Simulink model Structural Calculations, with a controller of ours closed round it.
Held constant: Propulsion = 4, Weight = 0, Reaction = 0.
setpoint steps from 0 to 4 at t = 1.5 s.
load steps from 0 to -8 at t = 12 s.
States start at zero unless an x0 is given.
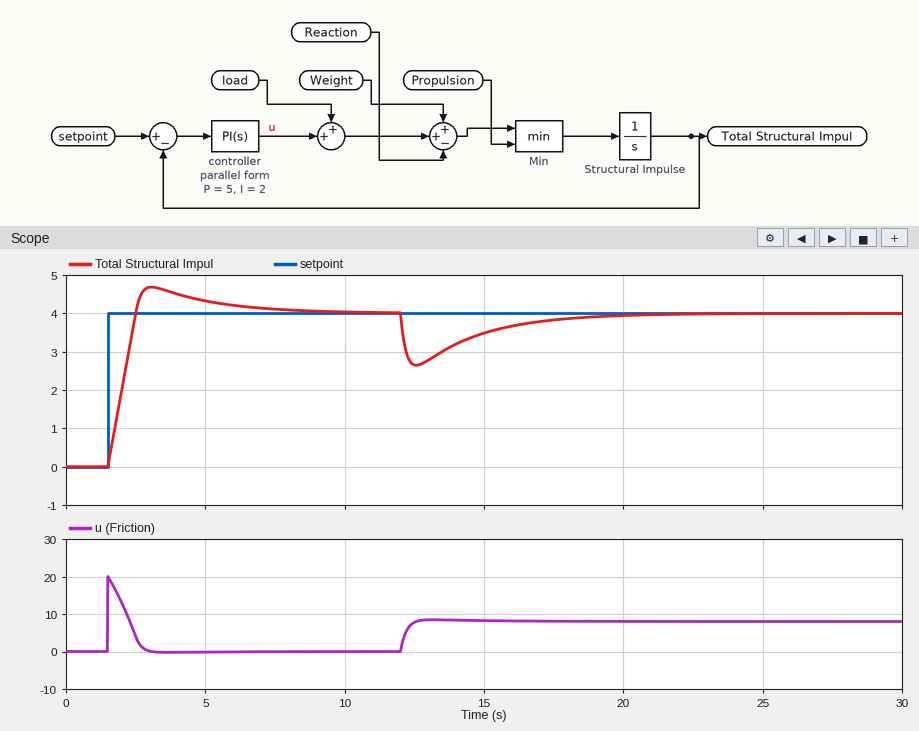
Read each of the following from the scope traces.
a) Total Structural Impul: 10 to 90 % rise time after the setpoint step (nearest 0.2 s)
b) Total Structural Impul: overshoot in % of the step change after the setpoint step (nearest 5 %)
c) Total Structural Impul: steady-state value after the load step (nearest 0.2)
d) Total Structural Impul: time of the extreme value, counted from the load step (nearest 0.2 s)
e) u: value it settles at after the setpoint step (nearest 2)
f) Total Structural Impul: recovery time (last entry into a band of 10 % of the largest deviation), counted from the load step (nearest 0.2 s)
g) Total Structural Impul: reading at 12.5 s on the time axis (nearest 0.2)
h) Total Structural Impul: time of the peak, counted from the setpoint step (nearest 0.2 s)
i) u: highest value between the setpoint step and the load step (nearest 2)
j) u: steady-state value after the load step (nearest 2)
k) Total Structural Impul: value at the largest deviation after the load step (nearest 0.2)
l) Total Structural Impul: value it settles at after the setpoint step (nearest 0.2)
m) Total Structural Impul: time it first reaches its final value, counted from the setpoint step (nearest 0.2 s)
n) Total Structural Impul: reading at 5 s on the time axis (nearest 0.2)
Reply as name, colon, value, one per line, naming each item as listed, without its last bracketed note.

Total Structural Impul: 10 to 90 % rise time after the setpoint step: 0.8 s
Total Structural Impul: overshoot in % of the step change after the setpoint step: 15 %
Total Structural Impul: steady-state value after the load step: 4.0
Total Structural Impul: time of the extreme value, counted from the load step: 0.6 s
u: value it settles at after the setpoint step: 0
Total Structural Impul: recovery time (last entry into a band of 10 % of the largest deviation), counted from the load step: 6.0 s
Total Structural Impul: reading at 12.5 s on the time axis: 2.6
Total Structural Impul: time of the peak, counted from the setpoint step: 1.6 s
u: highest value between the setpoint step and the load step: 20
u: steady-state value after the load step: 8
Total Structural Impul: value at the largest deviation after the load step: 2.6
Total Structural Impul: value it settles at after the setpoint step: 4.0
Total Structural Impul: time it first reaches its final value, counted from the setpoint step: 1.0 s
Total Structural Impul: reading at 5 s on the time axis: 4.4
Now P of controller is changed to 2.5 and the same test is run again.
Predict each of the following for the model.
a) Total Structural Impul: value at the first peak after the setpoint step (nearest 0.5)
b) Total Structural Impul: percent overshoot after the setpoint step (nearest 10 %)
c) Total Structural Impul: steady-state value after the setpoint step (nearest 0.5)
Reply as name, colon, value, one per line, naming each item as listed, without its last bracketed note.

Total Structural Impul: value at the first peak after the setpoint step: 5.0
Total Structural Impul: percent overshoot after the setpoint step: 30 %
Total Structural Impul: steady-state value after the setpoint step: 4.0
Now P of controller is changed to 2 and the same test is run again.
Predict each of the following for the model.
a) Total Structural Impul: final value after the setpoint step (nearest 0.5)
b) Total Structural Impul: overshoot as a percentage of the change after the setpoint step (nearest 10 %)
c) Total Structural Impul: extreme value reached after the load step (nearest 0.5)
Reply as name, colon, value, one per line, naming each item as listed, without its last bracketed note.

Total Structural Impul: final value after the setpoint step: 4.0
Total Structural Impul: overshoot as a percentage of the change after the setpoint step: 30 %
Total Structural Impul: extreme value reached after the load step: 1.5
